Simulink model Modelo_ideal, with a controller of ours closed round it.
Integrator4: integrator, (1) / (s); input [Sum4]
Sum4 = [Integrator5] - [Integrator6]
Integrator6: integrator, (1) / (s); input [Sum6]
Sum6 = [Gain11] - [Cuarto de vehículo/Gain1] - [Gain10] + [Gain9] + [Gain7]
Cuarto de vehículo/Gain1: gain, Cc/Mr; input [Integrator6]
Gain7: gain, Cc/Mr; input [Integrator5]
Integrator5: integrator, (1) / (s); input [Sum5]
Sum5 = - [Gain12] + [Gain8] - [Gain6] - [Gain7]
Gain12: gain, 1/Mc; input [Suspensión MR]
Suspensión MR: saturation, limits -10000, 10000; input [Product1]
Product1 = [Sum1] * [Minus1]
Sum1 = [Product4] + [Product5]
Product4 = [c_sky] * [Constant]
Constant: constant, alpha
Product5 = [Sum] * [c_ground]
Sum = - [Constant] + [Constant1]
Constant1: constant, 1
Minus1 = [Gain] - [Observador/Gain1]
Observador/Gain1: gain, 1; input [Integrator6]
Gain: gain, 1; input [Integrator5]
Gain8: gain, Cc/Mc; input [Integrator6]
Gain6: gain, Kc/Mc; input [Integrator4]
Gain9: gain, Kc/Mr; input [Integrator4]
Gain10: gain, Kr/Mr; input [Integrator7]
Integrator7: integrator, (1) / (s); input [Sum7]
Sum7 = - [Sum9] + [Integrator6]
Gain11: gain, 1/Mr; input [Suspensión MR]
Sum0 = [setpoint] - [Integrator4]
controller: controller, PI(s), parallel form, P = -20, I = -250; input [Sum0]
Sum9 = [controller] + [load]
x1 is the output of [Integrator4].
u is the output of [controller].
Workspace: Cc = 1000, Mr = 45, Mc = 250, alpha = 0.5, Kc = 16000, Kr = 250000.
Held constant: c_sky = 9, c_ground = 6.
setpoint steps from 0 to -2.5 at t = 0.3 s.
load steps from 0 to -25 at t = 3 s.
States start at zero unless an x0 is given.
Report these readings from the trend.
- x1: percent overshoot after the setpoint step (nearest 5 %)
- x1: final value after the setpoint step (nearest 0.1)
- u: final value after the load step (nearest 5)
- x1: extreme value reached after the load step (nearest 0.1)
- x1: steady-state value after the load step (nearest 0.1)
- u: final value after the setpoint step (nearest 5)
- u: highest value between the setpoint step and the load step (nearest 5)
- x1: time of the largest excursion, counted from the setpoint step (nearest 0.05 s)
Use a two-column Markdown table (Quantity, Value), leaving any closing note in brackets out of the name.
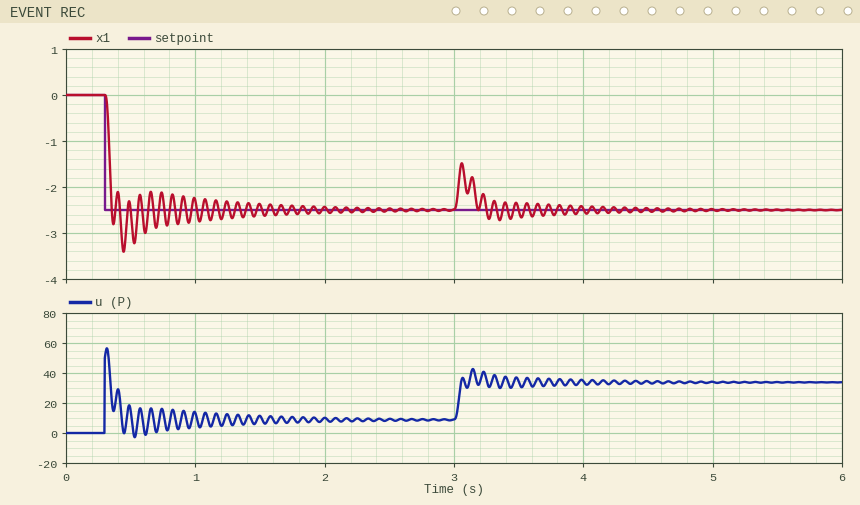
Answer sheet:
| Quantity | Value |
|---|---|
| x1: percent overshoot after the setpoint step | 35 % |
| x1: final value after the setpoint step | -2.5 |
| u: final value after the load step | 35 |
| x1: extreme value reached after the load step | -1.5 |
| x1: steady-state value after the load step | -2.5 |
| u: final value after the setpoint step | 10 |
| u: highest value between the setpoint step and the load step | 55 |
| x1: time of the largest excursion, counted from the setpoint step | 0.15 s |
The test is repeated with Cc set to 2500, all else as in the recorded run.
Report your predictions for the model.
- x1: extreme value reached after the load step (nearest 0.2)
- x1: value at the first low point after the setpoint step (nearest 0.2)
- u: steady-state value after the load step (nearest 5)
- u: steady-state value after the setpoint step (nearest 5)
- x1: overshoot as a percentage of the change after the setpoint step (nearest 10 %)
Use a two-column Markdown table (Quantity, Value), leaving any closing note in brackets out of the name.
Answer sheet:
| Quantity | Value |
|---|---|
| x1: extreme value reached after the load step | -1.6 |
| x1: value at the first low point after the setpoint step | -3.2 |
| u: steady-state value after the load step | 30 |
| u: steady-state value after the setpoint step | 5 |
| x1: overshoot as a percentage of the change after the setpoint step | 30 % |
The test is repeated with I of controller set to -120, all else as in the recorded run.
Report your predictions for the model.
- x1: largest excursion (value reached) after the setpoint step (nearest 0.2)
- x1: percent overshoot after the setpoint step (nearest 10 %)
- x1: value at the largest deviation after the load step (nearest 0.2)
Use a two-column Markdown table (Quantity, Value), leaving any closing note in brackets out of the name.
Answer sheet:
| Quantity | Value |
|---|---|
| x1: largest excursion (value reached) after the setpoint step | -3.0 |
| x1: percent overshoot after the setpoint step | 20 % |
| x1: value at the largest deviation after the load step | -1.4 |
